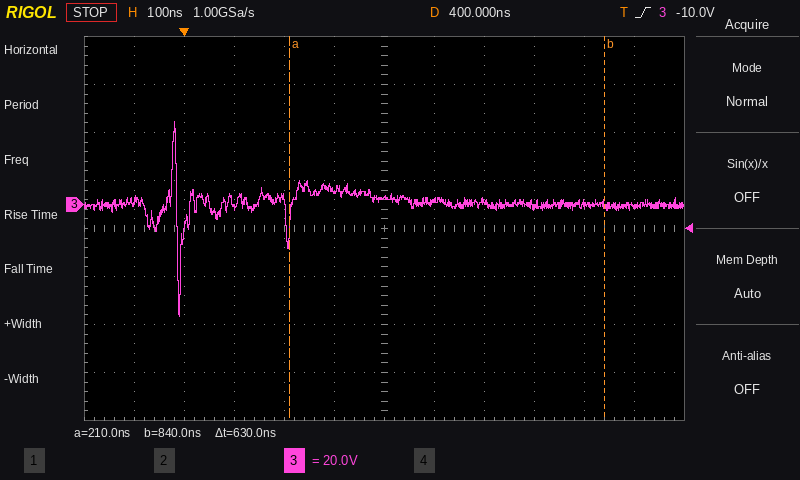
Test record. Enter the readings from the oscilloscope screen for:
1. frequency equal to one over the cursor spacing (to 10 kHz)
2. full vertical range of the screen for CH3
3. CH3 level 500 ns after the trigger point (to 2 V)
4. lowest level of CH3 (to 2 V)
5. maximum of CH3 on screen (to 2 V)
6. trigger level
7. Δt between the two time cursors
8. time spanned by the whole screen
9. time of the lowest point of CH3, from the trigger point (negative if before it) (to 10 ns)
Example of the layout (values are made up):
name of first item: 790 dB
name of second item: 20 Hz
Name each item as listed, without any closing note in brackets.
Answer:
frequency equal to one over the cursor spacing: 1.59 MHz
full vertical range of the screen for CH3: 160 V
CH3 level 500 ns after the trigger point: 2 V
lowest level of CH3: -46 V
maximum of CH3 on screen: 34 V
trigger level: -10.0 V
Δt between the two time cursors: 630 ns
time spanned by the whole screen: 1.2 µs
time of the lowest point of CH3, from the trigger point (negative if before it): -10 ns
